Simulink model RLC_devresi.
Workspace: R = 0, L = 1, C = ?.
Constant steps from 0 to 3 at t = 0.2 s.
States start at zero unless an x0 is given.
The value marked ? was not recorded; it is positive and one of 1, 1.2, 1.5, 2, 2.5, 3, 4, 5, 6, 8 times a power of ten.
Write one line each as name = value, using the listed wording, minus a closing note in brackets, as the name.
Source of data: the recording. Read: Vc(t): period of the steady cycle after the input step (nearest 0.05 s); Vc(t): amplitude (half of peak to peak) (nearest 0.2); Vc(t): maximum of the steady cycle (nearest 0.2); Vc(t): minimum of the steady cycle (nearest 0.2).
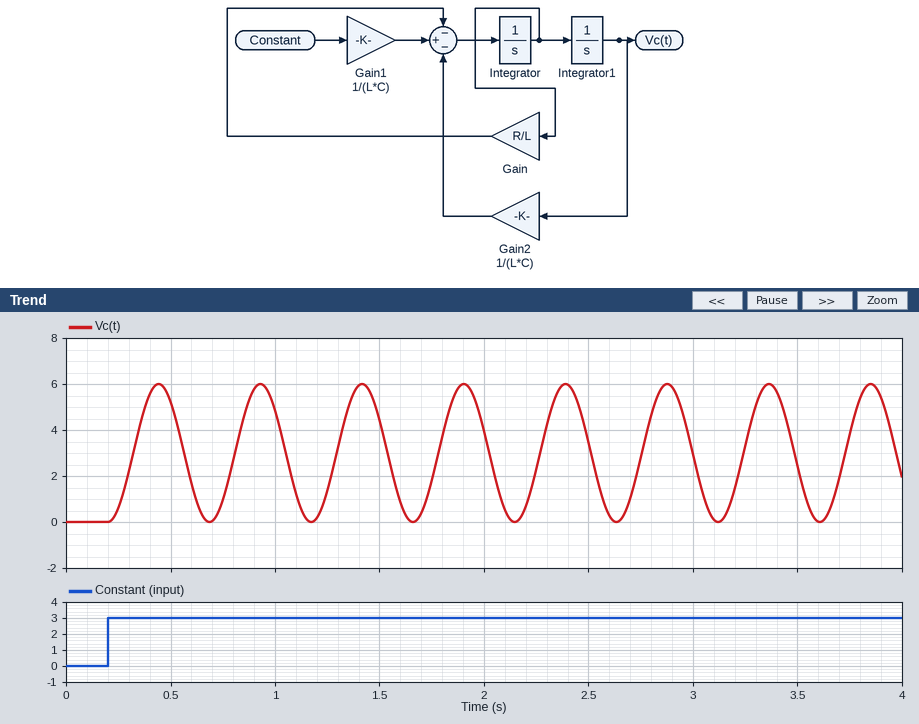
Vc(t): period of the steady cycle after the input step = 0.50 s
Vc(t): amplitude (half of peak to peak) = 3.0
Vc(t): maximum of the steady cycle = 6.0
Vc(t): minimum of the steady cycle = 0.0
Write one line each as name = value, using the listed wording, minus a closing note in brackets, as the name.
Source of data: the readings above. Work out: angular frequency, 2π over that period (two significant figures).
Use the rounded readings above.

angular frequency, 2π over that period = 13 rad/s
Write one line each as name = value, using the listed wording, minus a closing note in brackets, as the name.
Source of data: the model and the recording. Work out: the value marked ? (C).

the value marked ? = 0.006
